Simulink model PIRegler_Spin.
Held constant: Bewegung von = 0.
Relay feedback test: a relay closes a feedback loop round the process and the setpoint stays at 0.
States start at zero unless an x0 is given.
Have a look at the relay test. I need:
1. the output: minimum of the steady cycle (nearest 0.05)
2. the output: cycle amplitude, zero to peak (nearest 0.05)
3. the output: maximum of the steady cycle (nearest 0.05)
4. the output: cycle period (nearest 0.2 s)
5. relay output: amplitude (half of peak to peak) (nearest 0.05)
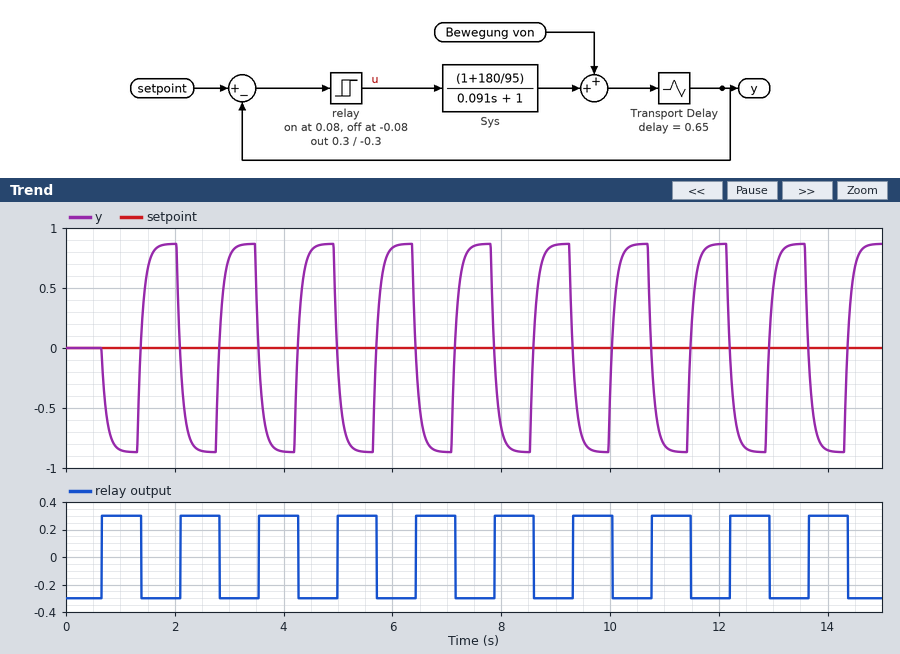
-0.85
0.85
0.85
1.4 s
0.30
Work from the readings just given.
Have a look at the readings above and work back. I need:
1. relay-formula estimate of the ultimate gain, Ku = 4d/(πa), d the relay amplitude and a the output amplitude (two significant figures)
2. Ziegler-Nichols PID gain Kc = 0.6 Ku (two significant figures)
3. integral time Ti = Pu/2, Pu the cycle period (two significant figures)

0.45
0.27
0.70 s
